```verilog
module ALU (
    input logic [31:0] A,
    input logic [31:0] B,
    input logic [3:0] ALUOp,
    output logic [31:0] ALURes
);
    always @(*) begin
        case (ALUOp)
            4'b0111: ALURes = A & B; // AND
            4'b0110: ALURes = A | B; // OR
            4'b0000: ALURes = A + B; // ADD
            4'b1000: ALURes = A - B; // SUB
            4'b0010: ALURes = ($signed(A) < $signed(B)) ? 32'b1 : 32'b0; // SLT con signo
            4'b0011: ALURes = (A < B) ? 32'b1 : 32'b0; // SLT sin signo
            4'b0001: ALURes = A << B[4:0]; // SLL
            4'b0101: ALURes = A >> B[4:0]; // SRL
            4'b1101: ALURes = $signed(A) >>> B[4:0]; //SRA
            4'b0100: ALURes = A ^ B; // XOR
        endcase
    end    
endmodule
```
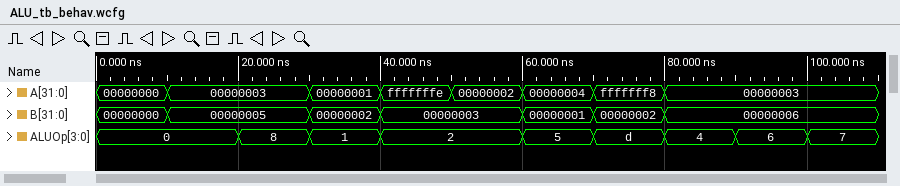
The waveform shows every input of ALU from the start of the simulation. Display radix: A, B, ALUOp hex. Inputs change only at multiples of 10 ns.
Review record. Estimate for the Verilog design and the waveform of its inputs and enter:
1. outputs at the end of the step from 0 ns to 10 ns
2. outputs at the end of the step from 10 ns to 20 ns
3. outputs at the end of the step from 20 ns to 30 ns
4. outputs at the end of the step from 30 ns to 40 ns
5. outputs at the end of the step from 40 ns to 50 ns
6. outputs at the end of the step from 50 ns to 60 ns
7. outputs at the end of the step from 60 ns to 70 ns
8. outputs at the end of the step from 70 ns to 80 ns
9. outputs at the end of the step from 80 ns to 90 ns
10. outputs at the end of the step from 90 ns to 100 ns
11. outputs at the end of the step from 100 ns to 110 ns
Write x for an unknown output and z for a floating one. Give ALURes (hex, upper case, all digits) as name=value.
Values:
ALURes=00000000
ALURes=00000008
ALURes=FFFFFFFE
ALURes=00000004
ALURes=00000001
ALURes=00000001
ALURes=00000002
ALURes=FFFFFFFE
ALURes=00000005
ALURes=00000007
ALURes=00000002
